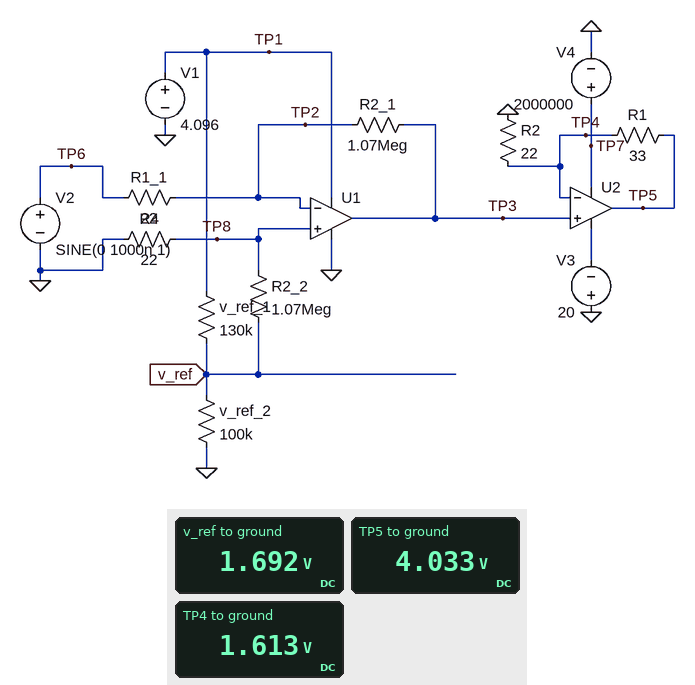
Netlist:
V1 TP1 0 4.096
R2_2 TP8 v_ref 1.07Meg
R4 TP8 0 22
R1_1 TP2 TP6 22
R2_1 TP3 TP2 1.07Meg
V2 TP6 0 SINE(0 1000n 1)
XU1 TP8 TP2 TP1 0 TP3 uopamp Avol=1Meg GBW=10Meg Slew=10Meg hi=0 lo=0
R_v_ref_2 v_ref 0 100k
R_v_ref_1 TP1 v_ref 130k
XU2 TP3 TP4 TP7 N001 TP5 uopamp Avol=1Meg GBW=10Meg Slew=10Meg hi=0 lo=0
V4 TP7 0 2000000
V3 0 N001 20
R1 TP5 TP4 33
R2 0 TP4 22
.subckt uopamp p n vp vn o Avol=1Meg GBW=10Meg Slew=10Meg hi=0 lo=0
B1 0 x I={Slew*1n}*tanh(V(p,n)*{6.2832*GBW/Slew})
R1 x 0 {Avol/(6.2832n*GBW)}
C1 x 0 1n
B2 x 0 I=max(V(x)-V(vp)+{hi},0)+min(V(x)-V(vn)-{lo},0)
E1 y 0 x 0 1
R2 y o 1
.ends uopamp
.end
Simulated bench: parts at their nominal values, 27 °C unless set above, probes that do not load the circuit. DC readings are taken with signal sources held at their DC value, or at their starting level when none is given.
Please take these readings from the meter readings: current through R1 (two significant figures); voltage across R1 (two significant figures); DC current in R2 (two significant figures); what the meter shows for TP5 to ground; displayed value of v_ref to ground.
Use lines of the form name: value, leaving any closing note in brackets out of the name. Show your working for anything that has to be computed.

current through R1: (4.033 V - 1.613 V) / 33 Ω = 73 mA
voltage across R1: 4.033 V - 1.613 V = 2.4 V
DC current in R2: (1.613 V) / 22 Ω = 73 mA
what the meter shows for TP5 to ground: 4.033 V
displayed value of v_ref to ground: 1.692 V
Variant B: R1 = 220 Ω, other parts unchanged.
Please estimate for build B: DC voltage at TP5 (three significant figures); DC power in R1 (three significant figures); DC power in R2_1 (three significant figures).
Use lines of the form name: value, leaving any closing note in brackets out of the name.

DC voltage at TP5: 17.7 V
DC power in R1: 1.18 W
DC power in R2_1: 2.43 µW
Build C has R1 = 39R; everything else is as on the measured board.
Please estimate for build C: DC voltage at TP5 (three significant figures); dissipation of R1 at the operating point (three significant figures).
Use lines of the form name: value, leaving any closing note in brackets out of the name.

DC voltage at TP5: 4.47 V
dissipation of R1 at the operating point: 210 mW
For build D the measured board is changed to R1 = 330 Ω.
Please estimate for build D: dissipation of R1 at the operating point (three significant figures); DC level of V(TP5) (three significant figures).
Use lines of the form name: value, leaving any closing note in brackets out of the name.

dissipation of R1 at the operating point: 1.77 W
DC level of V(TP5): 25.8 V
